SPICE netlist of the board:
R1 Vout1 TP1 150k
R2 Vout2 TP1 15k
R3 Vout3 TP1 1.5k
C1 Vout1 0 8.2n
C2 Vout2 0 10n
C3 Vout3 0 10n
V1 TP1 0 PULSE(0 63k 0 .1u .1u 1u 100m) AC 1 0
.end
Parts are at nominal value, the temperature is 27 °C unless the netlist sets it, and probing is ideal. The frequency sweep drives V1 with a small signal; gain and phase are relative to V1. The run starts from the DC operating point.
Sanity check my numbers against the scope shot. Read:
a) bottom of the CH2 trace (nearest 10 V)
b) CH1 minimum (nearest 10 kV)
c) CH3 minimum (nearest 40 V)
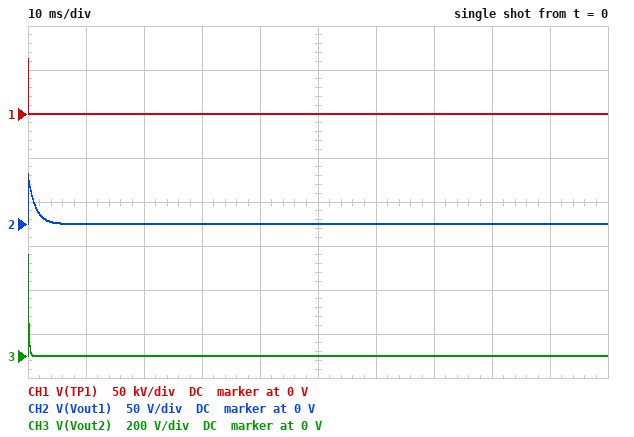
0 V
0 V
0 V
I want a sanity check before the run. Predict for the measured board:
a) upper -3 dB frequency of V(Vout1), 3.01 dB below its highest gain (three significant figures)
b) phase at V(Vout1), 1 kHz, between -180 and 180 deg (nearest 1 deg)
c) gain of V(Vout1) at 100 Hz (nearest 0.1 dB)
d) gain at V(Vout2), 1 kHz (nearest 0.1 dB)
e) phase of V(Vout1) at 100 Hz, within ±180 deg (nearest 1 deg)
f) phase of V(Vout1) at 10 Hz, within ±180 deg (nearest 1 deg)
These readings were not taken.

129 Hz
-83 deg
-2.0 dB
-2.8 dB
-38 deg
-4 deg
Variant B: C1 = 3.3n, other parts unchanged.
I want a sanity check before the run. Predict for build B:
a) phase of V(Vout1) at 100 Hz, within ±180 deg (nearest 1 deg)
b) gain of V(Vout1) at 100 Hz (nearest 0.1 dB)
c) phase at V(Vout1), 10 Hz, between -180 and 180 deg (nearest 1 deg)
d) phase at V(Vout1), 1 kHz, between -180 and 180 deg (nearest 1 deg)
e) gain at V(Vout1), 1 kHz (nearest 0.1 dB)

-17 deg
-0.4 dB
-2 deg
-72 deg
-10.3 dB
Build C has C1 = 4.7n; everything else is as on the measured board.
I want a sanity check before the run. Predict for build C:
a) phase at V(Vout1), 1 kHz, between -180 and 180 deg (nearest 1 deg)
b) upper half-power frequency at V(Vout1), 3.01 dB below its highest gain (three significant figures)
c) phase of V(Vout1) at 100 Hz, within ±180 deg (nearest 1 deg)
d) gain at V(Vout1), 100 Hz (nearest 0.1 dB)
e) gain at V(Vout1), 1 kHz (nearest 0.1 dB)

-77 deg
226 Hz
-24 deg
-0.8 dB
-13.1 dB
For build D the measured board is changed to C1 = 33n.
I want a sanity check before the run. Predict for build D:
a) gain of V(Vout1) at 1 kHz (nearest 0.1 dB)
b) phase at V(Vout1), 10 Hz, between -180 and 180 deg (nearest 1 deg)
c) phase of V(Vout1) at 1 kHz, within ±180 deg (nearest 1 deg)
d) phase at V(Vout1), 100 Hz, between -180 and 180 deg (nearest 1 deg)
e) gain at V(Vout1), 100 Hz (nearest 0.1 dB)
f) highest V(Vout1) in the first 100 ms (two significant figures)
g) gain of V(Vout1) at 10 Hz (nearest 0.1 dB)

-29.9 dB
-17 deg
-88 deg
-72 deg
-10.3 dB
14 V
-0.4 dB
